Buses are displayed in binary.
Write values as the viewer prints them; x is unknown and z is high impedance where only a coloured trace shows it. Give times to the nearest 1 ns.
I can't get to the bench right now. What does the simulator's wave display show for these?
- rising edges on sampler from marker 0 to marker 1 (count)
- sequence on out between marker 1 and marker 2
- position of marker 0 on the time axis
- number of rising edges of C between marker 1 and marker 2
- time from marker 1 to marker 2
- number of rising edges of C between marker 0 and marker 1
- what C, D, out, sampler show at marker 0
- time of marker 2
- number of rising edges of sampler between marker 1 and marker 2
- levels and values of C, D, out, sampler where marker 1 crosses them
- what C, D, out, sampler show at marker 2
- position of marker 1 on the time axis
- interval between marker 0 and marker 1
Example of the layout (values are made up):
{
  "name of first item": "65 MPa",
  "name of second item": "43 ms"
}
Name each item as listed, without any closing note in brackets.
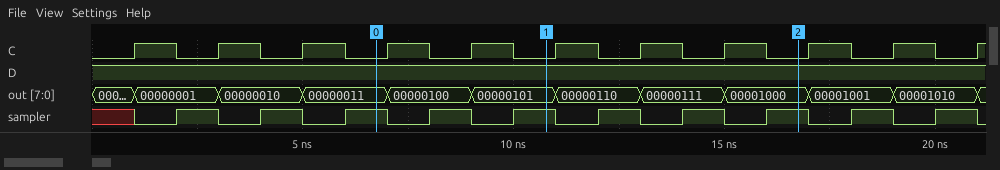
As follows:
{
  "rising edges on sampler from marker 0 to marker 1": "2",
  "sequence on out between marker 1 and marker 2": "00000101, 00000110, 00000111, 00001000",
  "position of marker 0 on the time axis": "7 ns",
  "number of rising edges of C between marker 1 and marker 2": "3",
  "time from marker 1 to marker 2": "6 ns",
  "number of rising edges of C between marker 0 and marker 1": "2",
  "what C, D, out, sampler show at marker 0": "C=0, D=1, out=00000011, sampler=1",
  "time of marker 2": "17 ns",
  "number of rising edges of sampler between marker 1 and marker 2": "3",
  "levels and values of C, D, out, sampler where marker 1 crosses them": "C=0, D=1, out=00000101, sampler=1",
  "what C, D, out, sampler show at marker 2": "C=0, D=1, out=00001000, sampler=1",
  "position of marker 1 on the time axis": "11 ns",
  "interval between marker 0 and marker 1": "4 ns"
}
